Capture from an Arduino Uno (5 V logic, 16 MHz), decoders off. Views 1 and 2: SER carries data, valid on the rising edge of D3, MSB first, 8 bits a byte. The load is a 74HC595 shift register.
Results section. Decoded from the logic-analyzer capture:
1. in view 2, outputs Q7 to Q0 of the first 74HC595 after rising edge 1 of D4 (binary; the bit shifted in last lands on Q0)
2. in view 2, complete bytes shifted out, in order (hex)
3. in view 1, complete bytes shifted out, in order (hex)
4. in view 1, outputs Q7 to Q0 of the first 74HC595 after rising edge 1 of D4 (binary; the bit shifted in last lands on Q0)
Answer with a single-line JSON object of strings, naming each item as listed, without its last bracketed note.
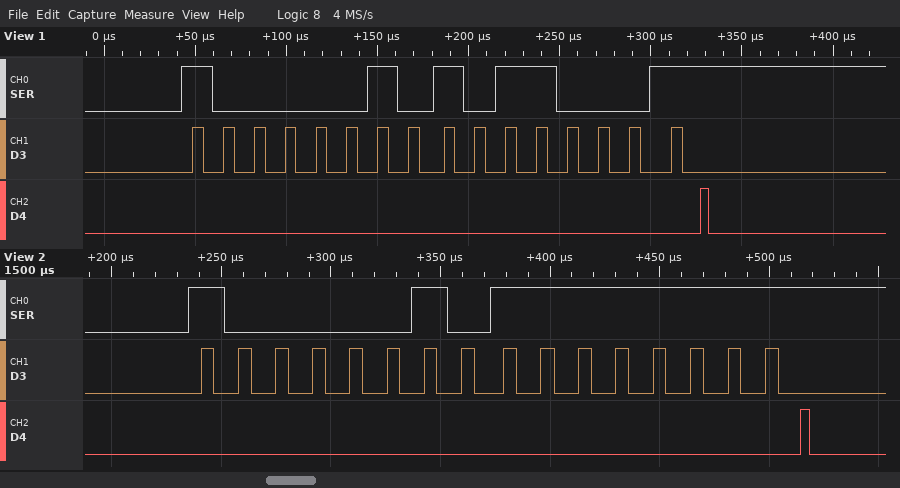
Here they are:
{"in view 2, outputs Q7 to Q0 of the first 74HC595 after rising edge 1 of D4": "11111111", "in view 2, complete bytes shifted out, in order": "82 FF", "in view 1, complete bytes shifted out, in order": "82 B1", "in view 1, outputs Q7 to Q0 of the first 74HC595 after rising edge 1 of D4": "10110001"}
